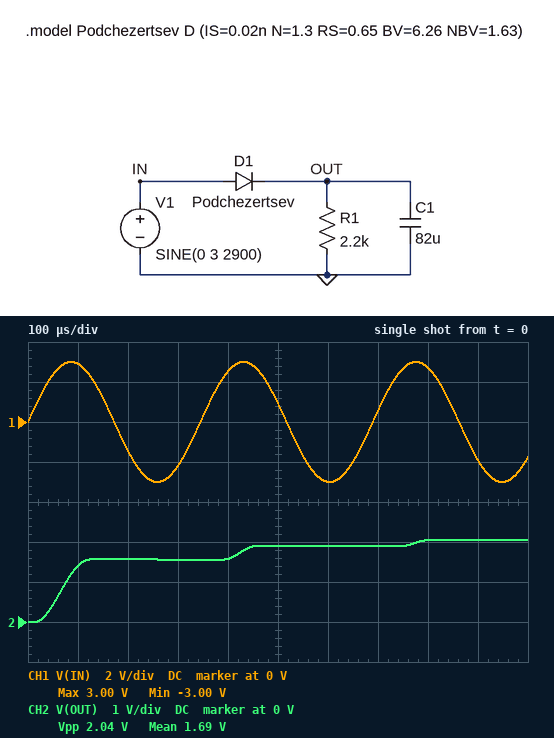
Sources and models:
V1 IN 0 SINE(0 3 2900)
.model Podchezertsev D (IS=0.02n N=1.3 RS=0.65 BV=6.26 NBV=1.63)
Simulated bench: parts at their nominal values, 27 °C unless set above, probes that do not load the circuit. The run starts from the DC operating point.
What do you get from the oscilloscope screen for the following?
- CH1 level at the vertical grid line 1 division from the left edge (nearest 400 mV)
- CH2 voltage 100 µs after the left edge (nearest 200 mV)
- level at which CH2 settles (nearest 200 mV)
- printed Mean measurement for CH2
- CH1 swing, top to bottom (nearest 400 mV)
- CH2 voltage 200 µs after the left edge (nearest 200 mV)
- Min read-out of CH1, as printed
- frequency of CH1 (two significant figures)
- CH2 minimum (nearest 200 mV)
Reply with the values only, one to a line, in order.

2.8 V
1.4 V
2.0 V
1.69 V
6.0 V
1.6 V
-3.00 V
2.9 kHz
0 V
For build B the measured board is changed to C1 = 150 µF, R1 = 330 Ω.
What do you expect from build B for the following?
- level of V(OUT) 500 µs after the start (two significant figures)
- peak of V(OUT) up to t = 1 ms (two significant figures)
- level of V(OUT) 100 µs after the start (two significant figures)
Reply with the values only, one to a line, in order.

1.6 V
1.8 V
960 mV
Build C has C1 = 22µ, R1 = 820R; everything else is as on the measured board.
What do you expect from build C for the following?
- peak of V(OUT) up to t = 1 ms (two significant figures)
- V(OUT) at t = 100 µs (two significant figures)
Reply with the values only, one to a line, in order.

2.2 V
2.1 V
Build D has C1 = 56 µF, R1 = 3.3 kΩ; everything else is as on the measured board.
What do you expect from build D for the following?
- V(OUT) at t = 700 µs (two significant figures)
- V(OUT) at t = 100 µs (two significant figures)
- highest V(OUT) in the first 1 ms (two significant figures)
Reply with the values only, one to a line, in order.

2.0 V
1.7 V
2.1 V
